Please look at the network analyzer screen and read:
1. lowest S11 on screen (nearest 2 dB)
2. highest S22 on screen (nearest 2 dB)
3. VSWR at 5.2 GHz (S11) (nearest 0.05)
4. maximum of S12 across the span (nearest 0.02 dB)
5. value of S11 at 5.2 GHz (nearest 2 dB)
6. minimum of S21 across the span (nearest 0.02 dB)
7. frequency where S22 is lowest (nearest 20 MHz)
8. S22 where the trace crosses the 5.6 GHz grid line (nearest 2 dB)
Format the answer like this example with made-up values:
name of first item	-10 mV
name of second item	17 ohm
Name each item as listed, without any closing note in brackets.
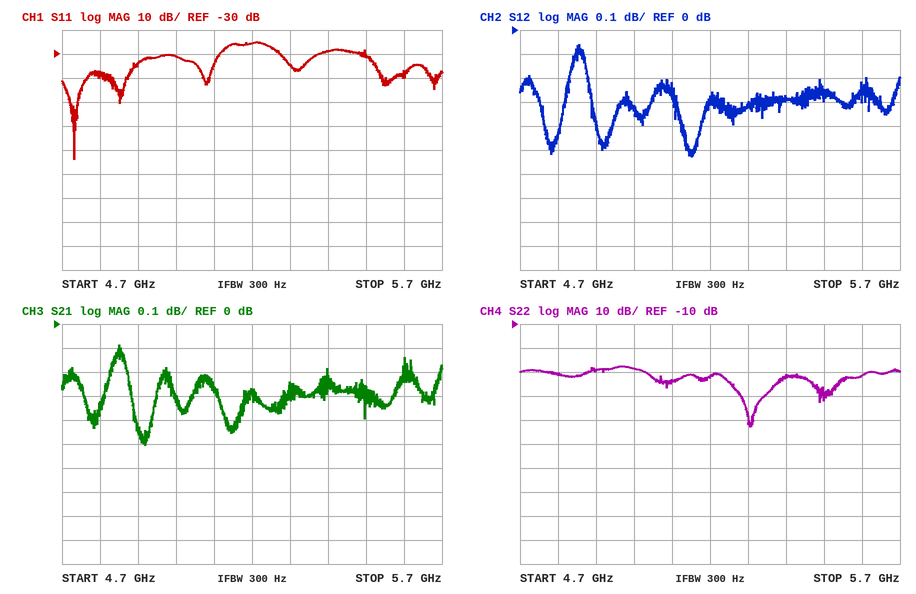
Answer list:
lowest S11 on screen	-74 dB
highest S22 on screen	-28 dB
VSWR at 5.2 GHz (S11)	1.10
maximum of S12 across the span	-0.06 dB
value of S11 at 5.2 GHz	-26 dB
minimum of S21 across the span	-0.50 dB
frequency where S22 is lowest	5.30 GHz
S22 where the trace crosses the 5.6 GHz grid line	-32 dB
